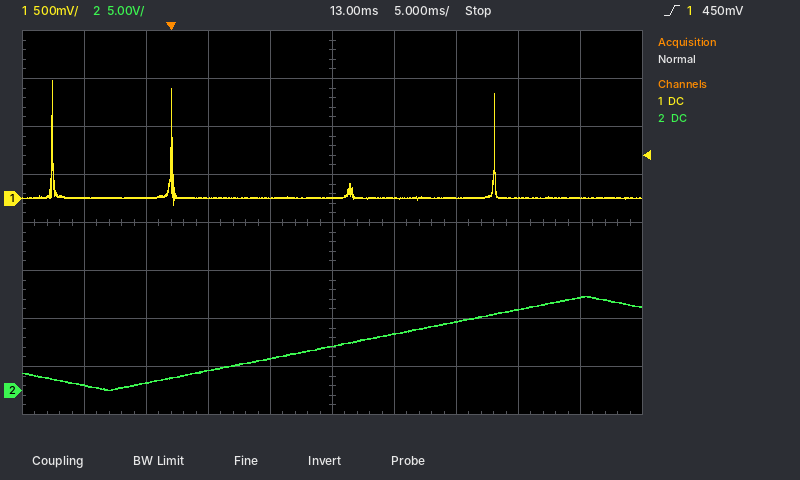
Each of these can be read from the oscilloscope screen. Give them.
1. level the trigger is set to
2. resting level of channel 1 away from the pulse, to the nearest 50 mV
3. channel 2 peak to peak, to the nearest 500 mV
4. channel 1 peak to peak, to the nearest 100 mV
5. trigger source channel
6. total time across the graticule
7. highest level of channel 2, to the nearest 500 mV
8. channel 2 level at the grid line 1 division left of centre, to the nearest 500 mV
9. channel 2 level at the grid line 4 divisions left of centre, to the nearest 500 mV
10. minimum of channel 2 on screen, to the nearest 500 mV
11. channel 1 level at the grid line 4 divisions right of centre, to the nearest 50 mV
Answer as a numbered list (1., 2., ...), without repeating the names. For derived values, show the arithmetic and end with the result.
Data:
1. 450 mV
2. 0 mV
3. 10.0 V − (0.0 V) = 10.0 V
4. 1.30 V
5. channel 1
6. 50 ms
7. 10.0 V
8. 3.5 V
9. 500 mV
10. 0.0 V
11. 0 mV
